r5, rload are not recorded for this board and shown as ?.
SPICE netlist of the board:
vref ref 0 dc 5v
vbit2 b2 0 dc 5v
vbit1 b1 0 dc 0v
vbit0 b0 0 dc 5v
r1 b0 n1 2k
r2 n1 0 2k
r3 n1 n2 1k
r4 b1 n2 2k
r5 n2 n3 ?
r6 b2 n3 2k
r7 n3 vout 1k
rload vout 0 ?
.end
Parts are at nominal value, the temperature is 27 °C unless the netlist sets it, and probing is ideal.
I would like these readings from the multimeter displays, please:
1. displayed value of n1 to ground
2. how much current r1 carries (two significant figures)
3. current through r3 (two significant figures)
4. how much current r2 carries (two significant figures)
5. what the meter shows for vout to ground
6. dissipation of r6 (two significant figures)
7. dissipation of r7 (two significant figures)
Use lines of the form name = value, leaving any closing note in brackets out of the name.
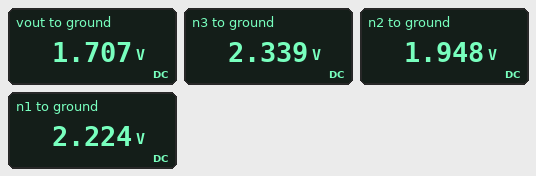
displayed value of n1 to ground = 2.224 V
how much current r1 carries = 1.4 mA
current through r3 = 280 µA
how much current r2 carries = 1.1 mA
what the meter shows for vout to ground = 1.707 V
dissipation of r6 = 3.5 mW
dissipation of r7 = 400 µW
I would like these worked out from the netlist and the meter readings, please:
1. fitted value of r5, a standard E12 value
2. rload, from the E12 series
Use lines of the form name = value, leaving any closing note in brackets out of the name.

fitted value of r5, a standard E12 value = 560 Ω
rload, from the E12 series = 2.7 kΩ
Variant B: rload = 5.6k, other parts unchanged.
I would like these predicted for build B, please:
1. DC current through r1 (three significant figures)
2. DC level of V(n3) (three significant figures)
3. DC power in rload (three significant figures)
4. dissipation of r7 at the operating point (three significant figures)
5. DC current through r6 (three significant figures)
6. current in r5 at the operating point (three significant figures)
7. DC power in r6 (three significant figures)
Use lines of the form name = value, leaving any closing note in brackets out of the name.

DC current through r1 = 1.35 mA
DC level of V(n3) = 2.55 V
DC power in rload = 839 µW
dissipation of r7 at the operating point = 150 µW
DC current through r6 = 1.22 mA
current in r5 at the operating point = 836 µA
DC power in r6 = 2.99 mW
